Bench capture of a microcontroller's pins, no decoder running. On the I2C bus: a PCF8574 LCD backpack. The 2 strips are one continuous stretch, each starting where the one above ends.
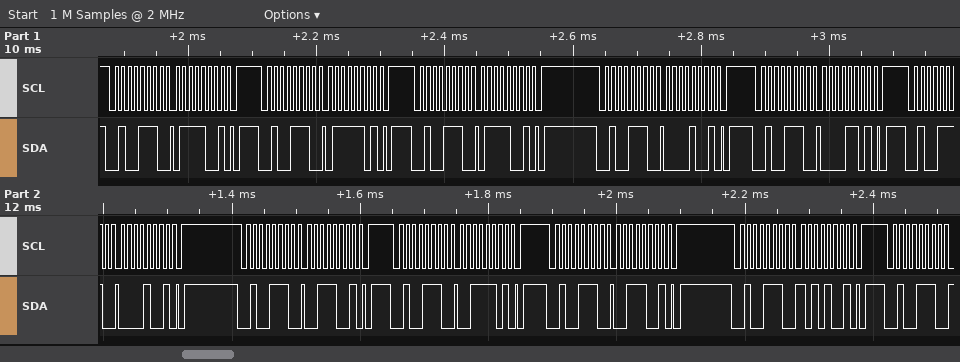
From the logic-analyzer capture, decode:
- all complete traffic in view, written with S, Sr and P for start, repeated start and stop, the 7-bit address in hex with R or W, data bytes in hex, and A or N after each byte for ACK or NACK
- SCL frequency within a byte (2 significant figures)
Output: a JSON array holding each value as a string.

["S 27W A 79 A P S 27W A 7D A P S 27W A 79 A P S 27W A 09 A P S 27W A 0D A P S 27W A 09 A P S 27W A 39 A P S 27W A 3D A P S 27W A 39 A P S 27W A A9 A P S 27W A", "100 kHz"]
